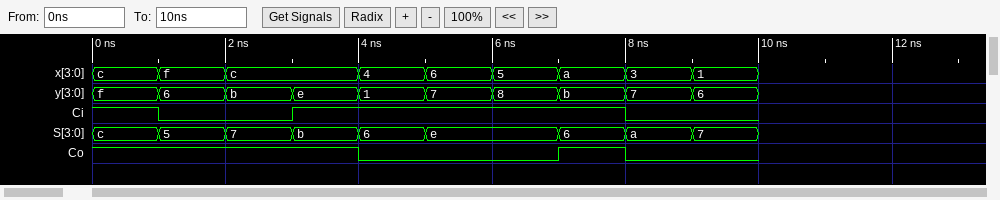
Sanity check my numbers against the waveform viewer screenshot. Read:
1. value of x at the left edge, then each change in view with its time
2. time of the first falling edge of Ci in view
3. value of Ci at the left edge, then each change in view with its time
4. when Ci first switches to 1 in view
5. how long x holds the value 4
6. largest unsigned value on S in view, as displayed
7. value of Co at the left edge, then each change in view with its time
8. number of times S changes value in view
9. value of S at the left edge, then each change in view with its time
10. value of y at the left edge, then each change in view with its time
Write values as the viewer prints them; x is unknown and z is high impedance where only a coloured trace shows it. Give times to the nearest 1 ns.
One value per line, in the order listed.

c, f at 1 ns, c at 2 ns, 4 at 4 ns, 6 at 5 ns, 5 at 6 ns, a at 7 ns, 3 at 8 ns, 1 at 9 ns
1 ns
1, 0 at 1 ns, 1 at 3 ns, 0 at 8 ns
3 ns
1 ns
e
1, 0 at 4 ns, 1 at 7 ns, 0 at 8 ns
8
c, 5 at 1 ns, 7 at 2 ns, b at 3 ns, 6 at 4 ns, e at 5 ns, 6 at 7 ns, a at 8 ns, 7 at 9 ns
f, 6 at 1 ns, b at 2 ns, e at 3 ns, 1 at 4 ns, 7 at 5 ns, 8 at 6 ns, b at 7 ns, 7 at 8 ns, 6 at 9 ns
